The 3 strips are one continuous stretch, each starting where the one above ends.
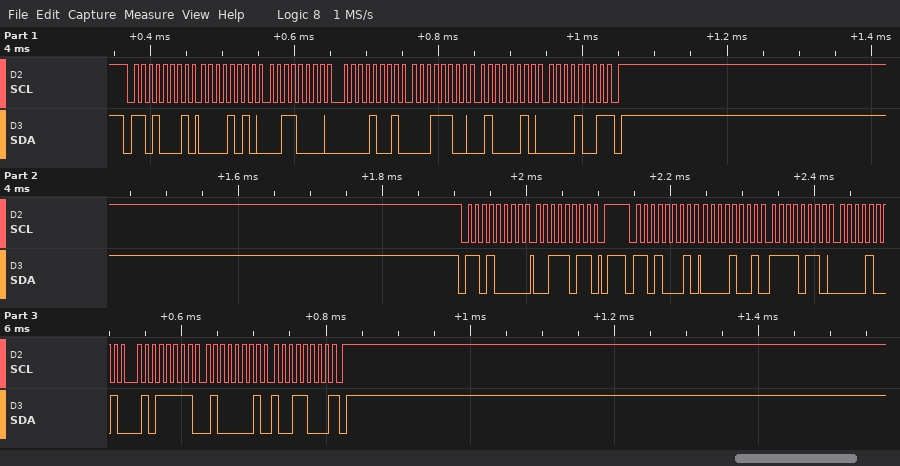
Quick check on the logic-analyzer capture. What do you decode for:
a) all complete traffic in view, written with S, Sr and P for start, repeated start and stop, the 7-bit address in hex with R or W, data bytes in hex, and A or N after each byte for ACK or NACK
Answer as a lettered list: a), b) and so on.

a) S 68R A 0A A 30 A 09 A 1C A 42 A 09 N P S 68W A 3B A P S 68R A 09 A F6 A 09 A 5F A 41 A 98 N P
